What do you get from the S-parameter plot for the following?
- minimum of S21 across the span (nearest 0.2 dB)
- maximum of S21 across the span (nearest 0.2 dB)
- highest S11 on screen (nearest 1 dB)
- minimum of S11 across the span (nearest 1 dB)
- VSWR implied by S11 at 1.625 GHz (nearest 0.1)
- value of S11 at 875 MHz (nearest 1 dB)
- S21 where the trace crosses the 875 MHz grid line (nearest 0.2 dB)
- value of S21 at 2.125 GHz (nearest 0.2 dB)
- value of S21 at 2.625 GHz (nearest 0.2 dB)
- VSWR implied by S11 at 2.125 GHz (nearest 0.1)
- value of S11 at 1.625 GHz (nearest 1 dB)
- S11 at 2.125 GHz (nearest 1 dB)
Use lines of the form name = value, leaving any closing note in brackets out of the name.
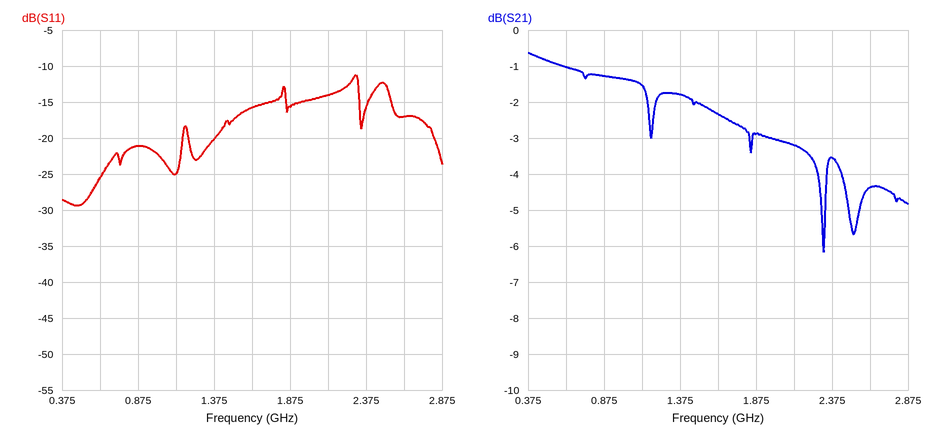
minimum of S21 across the span = -6.2 dB
maximum of S21 across the span = -0.6 dB
highest S11 on screen = -11 dB
minimum of S11 across the span = -29 dB
VSWR implied by S11 at 1.625 GHz = 1.4
value of S11 at 875 MHz = -21 dB
S21 where the trace crosses the 875 MHz grid line = -1.2 dB
value of S21 at 2.125 GHz = -3.2 dB
value of S21 at 2.625 GHz = -4.4 dB
VSWR implied by S11 at 2.125 GHz = 1.5
value of S11 at 1.625 GHz = -16 dB
S11 at 2.125 GHz = -14 dB
